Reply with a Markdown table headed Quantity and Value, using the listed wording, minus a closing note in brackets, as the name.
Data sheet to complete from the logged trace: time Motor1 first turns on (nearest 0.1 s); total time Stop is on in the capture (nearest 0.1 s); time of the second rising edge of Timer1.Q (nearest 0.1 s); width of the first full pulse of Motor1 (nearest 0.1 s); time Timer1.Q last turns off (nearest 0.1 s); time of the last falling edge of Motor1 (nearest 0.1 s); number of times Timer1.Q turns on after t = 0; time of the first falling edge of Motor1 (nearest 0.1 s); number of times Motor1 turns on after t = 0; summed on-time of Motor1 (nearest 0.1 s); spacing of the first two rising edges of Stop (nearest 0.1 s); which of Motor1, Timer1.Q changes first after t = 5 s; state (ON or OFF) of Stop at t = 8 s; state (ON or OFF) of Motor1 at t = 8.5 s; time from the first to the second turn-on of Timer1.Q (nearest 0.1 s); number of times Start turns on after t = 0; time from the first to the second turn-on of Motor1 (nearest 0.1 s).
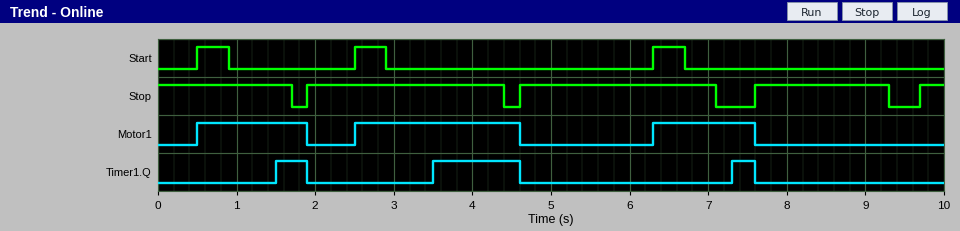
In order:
| Quantity | Value |
|---|---|
| time Motor1 first turns on | 0.5 s |
| total time Stop is on in the capture | 8.7 s |
| time of the second rising edge of Timer1.Q | 3.5 s |
| width of the first full pulse of Motor1 | 1.4 s |
| time Timer1.Q last turns off | 7.6 s |
| time of the last falling edge of Motor1 | 7.6 s |
| number of times Timer1.Q turns on after t = 0 | 3 |
| time of the first falling edge of Motor1 | 1.9 s |
| number of times Motor1 turns on after t = 0 | 3 |
| summed on-time of Motor1 | 4.8 s |
| spacing of the first two rising edges of Stop | 2.7 s |
| which of Motor1, Timer1.Q changes first after t = 5 s | Motor1 |
| state (ON or OFF) of Stop at t = 8 s | ON |
| state (ON or OFF) of Motor1 at t = 8.5 s | OFF |
| time from the first to the second turn-on of Timer1.Q | 2.0 s |
| number of times Start turns on after t = 0 | 3 |
| time from the first to the second turn-on of Motor1 | 2.0 s |
